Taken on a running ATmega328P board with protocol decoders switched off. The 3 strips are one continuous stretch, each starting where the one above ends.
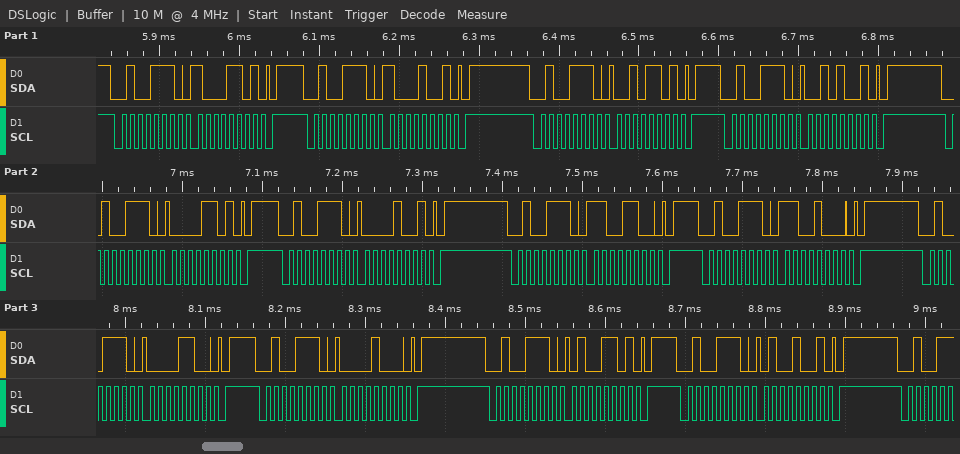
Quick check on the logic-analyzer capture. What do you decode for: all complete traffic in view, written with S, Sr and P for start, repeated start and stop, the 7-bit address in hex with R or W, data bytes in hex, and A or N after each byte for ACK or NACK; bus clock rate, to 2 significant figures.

S 27W A 8D A P S 27W A 89 A P S 27W A 2D A P S 27W A 29 A P S 27W A 0D A P S 27W A 09 A P S 27W A CC A P S 27W A C8 A P S 27W A 0C A P S 27W A 08 A P S 27W A 4D A P S 27W A 49 A P
100 kHz
